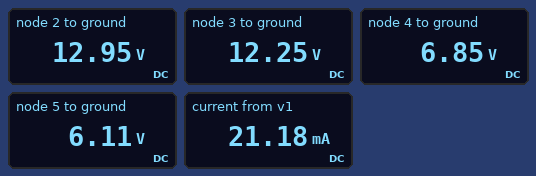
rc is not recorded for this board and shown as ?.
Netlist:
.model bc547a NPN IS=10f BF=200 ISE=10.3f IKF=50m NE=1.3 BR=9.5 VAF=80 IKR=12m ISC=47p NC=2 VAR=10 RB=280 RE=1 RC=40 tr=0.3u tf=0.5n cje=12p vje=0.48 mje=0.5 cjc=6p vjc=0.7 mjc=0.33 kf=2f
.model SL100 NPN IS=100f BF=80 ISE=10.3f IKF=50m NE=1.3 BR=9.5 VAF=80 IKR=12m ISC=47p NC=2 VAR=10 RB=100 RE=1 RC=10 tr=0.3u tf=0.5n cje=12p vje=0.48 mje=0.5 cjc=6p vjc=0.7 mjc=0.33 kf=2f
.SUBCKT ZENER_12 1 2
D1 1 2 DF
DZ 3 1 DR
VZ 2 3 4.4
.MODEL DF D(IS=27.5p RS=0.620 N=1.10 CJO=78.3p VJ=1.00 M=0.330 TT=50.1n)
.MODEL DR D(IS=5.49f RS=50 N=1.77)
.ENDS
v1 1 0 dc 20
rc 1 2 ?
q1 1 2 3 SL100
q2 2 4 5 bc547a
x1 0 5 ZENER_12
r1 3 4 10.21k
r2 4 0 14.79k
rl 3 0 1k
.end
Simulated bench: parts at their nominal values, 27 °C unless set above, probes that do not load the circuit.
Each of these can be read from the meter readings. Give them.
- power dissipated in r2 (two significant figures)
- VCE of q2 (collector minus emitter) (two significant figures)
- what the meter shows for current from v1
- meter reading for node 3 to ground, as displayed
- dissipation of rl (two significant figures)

3.2 mW
6.8 V
21.18 mA
12.25 V
150 mW
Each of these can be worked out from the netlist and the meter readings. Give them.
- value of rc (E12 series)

820 Ω
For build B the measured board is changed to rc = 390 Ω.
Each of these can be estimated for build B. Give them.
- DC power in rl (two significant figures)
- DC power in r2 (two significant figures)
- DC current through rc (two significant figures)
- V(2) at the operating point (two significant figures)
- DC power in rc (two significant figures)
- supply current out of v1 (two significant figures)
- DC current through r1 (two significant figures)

180 mW
3.5 mW
15 mA
14 V
87 mW
29 mA
610 µA
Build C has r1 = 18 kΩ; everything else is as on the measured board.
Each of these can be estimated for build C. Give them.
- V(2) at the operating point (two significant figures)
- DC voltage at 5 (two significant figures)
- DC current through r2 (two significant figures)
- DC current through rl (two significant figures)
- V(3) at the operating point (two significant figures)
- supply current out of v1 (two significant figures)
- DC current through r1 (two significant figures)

16 V
5.9 V
450 µA
15 mA
15 V
20 mA
480 µA
